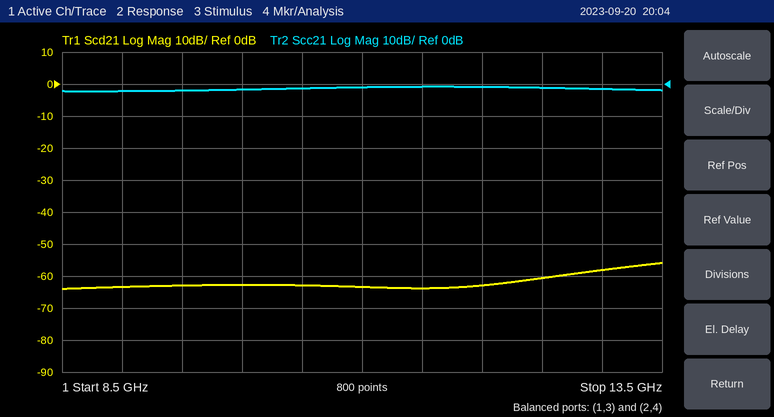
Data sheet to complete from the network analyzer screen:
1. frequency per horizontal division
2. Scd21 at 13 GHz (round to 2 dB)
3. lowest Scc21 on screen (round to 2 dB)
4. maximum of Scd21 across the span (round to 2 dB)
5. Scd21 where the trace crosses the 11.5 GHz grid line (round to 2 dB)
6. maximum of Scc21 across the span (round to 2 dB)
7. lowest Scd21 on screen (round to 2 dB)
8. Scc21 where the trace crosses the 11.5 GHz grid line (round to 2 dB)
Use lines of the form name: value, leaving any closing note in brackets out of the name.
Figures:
frequency per horizontal division: 500 MHz
Scd21 at 13 GHz: -58 dB
lowest Scc21 on screen: -2 dB
maximum of Scd21 across the span: -56 dB
Scd21 where the trace crosses the 11.5 GHz grid line: -64 dB
maximum of Scc21 across the span: 0 dB
lowest Scd21 on screen: -64 dB
Scc21 where the trace crosses the 11.5 GHz grid line: 0 dB
